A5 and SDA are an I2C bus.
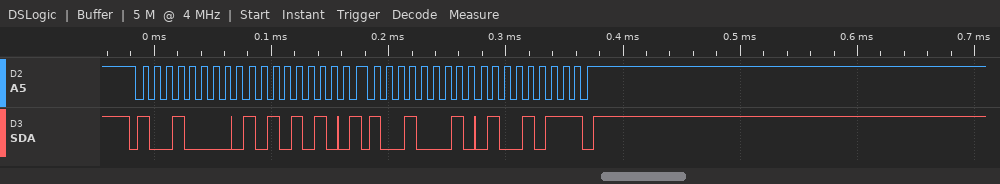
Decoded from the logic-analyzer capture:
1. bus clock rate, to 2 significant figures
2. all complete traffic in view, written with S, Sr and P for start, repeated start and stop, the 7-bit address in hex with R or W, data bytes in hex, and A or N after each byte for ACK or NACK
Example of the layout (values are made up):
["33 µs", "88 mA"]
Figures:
["100 kHz", "S 48W A AA A Sr 48R A 4B N P"]
